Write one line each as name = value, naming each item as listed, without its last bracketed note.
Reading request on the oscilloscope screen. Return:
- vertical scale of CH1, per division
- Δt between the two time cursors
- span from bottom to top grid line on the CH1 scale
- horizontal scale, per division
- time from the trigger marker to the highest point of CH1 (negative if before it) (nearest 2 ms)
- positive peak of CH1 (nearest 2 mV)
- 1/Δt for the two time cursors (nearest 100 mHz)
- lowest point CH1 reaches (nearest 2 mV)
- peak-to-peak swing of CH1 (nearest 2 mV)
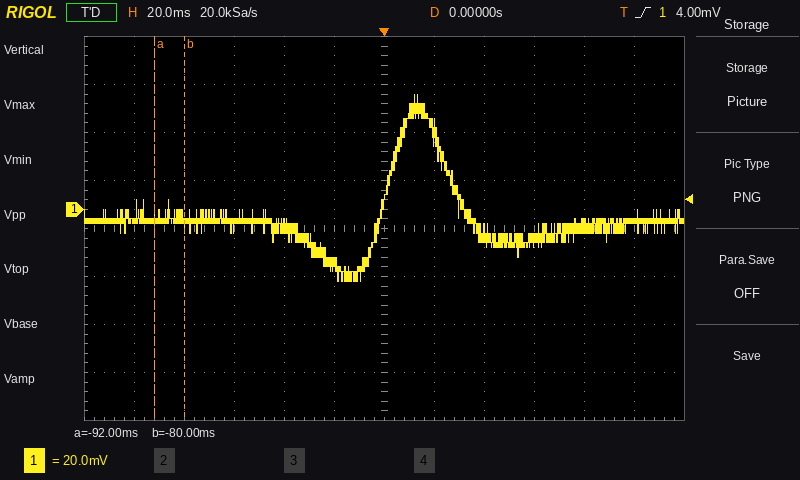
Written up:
vertical scale of CH1, per division = 20 mV
Δt between the two time cursors = 12 ms
span from bottom to top grid line on the CH1 scale = 160 mV
horizontal scale, per division = 20 ms
time from the trigger marker to the highest point of CH1 (negative if before it) = +12 ms
positive peak of CH1 = 48 mV
1/Δt for the two time cursors = 83.3 Hz
lowest point CH1 reaches = -30 mV
peak-to-peak swing of CH1 = 78 mV
